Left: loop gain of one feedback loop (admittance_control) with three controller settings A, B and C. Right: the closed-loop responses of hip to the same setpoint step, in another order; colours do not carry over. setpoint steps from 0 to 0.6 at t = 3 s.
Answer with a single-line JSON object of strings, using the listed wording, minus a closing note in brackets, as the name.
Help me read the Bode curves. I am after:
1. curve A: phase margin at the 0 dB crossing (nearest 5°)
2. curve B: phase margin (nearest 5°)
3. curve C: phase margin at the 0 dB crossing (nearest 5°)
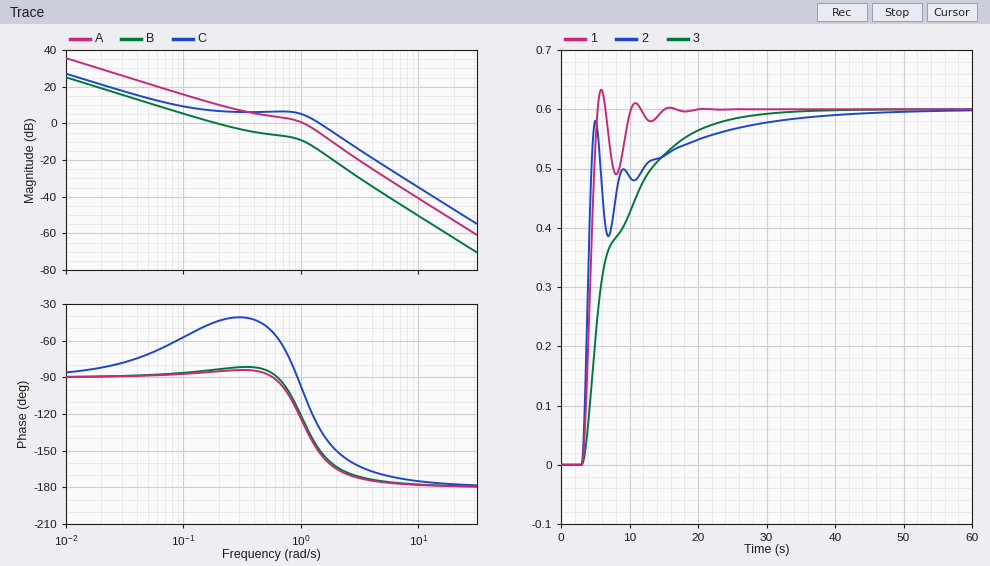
{"curve A: phase margin at the 0 dB crossing": "50°", "curve B: phase margin": "95°", "curve C: phase margin at the 0 dB crossing": "50°"}
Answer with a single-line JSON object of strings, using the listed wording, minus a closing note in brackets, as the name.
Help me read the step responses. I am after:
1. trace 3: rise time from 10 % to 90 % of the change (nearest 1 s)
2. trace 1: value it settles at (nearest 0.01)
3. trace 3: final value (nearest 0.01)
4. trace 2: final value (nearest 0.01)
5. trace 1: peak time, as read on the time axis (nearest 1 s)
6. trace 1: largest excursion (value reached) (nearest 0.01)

{"trace 3: rise time from 10 % to 90 % of the change": "13 s", "trace 1: value it settles at": "0.60", "trace 3: final value": "0.60", "trace 2: final value": "0.60", "trace 1: peak time, as read on the time axis": "6 s", "trace 1: largest excursion (value reached)": "0.63"}
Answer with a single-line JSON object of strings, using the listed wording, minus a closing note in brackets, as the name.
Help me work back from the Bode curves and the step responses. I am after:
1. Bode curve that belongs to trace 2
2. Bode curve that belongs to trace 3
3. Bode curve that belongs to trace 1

{"Bode curve that belongs to trace 2": "C", "Bode curve that belongs to trace 3": "B", "Bode curve that belongs to trace 1": "A"}
